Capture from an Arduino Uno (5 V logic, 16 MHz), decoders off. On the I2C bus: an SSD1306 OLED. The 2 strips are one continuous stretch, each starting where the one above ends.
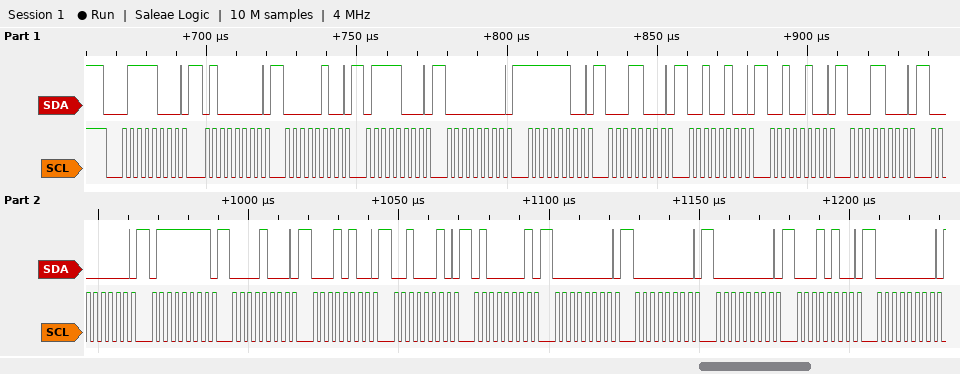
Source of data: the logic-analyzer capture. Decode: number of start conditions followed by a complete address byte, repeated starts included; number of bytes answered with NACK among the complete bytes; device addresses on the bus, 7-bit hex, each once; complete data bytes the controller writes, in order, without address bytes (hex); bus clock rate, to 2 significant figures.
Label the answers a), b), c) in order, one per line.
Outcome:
a) 1
b) 0
c) 0x3C
d) 40 04 78 00 FC 18 24 24 18 00 7F 08 14 22 41 00 00 00 14 00
e) 400 kHz
